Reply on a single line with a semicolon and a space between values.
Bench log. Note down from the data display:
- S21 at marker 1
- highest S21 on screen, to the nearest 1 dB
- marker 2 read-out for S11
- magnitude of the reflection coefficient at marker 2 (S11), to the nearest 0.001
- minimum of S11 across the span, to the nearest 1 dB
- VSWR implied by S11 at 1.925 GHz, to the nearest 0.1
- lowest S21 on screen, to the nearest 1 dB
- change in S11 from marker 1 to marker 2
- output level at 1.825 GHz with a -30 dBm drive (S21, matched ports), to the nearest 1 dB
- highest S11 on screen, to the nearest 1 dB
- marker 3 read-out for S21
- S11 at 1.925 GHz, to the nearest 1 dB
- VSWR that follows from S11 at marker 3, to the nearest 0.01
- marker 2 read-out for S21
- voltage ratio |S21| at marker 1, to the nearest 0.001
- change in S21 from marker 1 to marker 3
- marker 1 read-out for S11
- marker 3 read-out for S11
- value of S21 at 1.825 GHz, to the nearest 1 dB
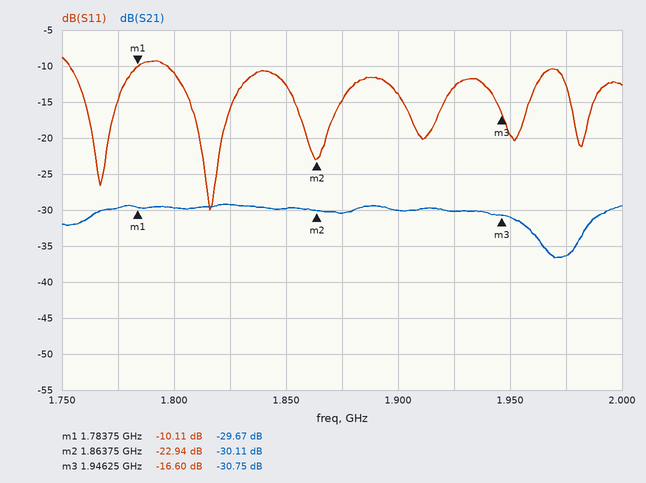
-29.67 dB; -29 dB; -22.94 dB; 0.071; -30 dB; 1.6; -37 dB; -12.83 dB; -59 dBm; -9 dB; -30.75 dB; -13 dB; 1.35; -30.11 dB; 0.033; -1.08 dB; -10.11 dB; -16.60 dB; -29 dB
